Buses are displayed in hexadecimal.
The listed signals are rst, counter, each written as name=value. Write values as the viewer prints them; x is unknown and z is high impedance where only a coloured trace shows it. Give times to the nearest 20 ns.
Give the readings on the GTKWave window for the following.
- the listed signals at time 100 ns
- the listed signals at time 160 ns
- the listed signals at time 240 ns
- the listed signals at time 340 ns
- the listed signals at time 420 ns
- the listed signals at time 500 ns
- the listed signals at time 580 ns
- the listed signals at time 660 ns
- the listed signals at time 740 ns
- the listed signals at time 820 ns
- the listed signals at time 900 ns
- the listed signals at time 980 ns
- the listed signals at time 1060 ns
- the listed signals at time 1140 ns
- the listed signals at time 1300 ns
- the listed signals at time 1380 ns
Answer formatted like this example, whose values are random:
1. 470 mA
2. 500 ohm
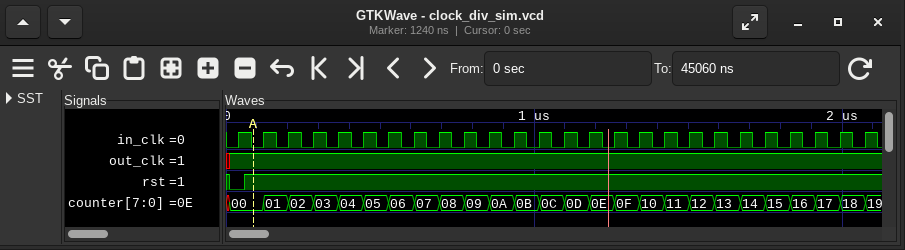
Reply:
1. rst=1, counter=00
2. rst=1, counter=01
3. rst=1, counter=02
4. rst=1, counter=03
5. rst=1, counter=04
6. rst=1, counter=05
7. rst=1, counter=06
8. rst=1, counter=07
9. rst=1, counter=08
10. rst=1, counter=09
11. rst=1, counter=0A
12. rst=1, counter=0B
13. rst=1, counter=0C
14. rst=1, counter=0D
15. rst=1, counter=0F
16. rst=1, counter=10
